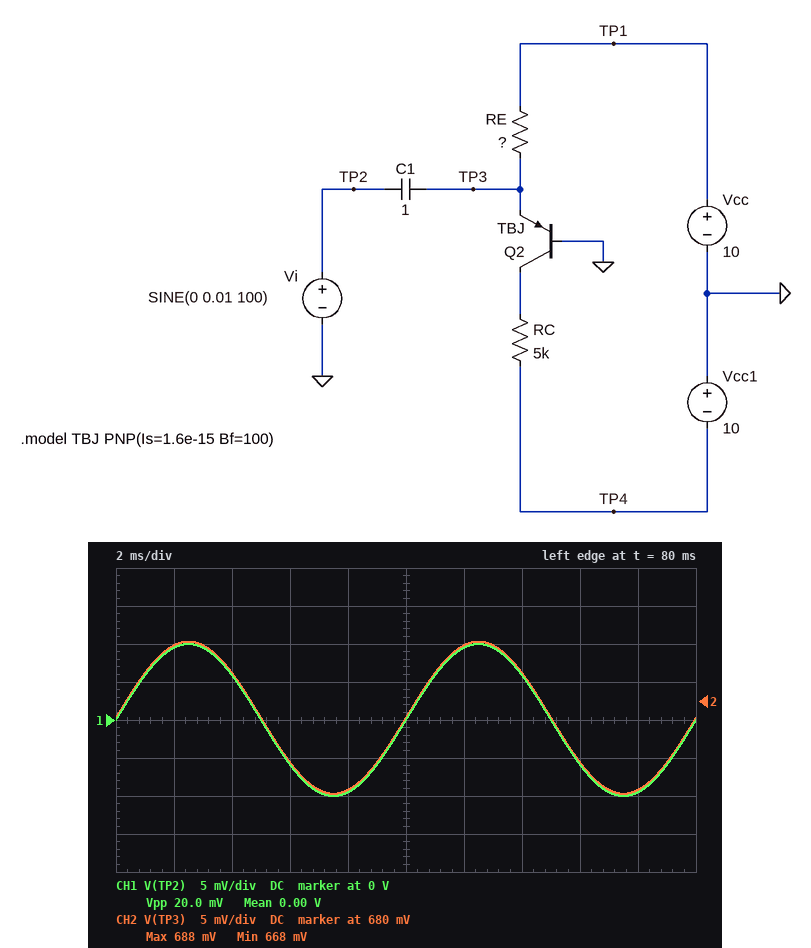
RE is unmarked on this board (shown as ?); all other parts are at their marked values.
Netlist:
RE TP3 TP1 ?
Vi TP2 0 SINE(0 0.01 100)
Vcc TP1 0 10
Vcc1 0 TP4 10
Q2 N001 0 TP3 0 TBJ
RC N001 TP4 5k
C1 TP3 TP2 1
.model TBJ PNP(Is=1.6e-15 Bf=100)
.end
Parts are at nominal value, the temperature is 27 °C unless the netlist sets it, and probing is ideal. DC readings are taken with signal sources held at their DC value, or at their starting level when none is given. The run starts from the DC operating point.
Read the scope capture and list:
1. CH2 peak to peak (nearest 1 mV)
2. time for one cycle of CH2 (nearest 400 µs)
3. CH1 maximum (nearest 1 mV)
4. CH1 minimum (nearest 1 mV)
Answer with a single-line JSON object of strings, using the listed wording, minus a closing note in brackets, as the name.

{"CH2 peak to peak": "20 mV", "time for one cycle of CH2": "10.0 ms", "CH1 maximum": "10 mV", "CH1 minimum": "-10 mV"}
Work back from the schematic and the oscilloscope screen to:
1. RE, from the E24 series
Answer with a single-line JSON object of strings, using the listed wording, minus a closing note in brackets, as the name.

{"RE, from the E24 series": "24 kΩ"}
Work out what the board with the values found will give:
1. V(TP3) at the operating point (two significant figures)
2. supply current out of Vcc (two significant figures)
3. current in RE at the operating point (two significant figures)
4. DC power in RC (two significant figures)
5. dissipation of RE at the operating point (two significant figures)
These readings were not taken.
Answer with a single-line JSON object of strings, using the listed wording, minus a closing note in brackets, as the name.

{"V(TP3) at the operating point": "680 mV", "supply current out of Vcc": "390 µA", "current in RE at the operating point": "390 µA", "DC power in RC": "740 µW", "dissipation of RE at the operating point": "3.6 mW"}
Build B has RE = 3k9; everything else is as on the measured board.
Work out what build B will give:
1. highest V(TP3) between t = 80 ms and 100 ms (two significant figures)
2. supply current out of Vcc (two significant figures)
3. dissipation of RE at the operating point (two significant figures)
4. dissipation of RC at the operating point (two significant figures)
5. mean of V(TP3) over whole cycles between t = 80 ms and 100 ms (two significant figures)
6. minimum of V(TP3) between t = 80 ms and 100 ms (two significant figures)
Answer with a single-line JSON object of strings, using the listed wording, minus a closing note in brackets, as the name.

{"highest V(TP3) between t = 80 ms and 100 ms": "740 mV", "supply current out of Vcc": "2.4 mA", "dissipation of RE at the operating point": "22 mW", "dissipation of RC at the operating point": "23 mW", "mean of V(TP3) over whole cycles between t = 80 ms and 100 ms": "730 mV", "minimum of V(TP3) between t = 80 ms and 100 ms": "720 mV"}
